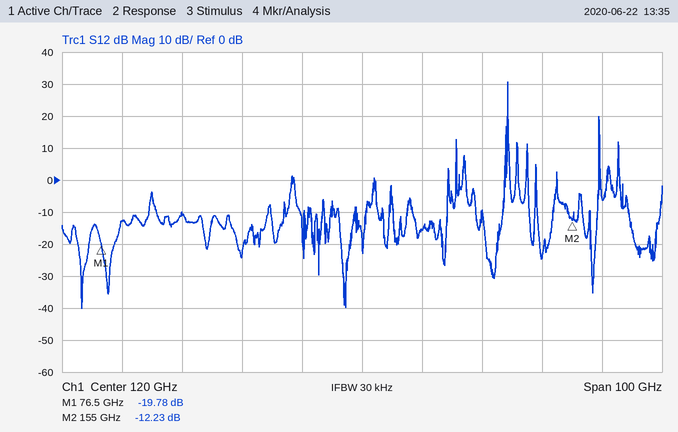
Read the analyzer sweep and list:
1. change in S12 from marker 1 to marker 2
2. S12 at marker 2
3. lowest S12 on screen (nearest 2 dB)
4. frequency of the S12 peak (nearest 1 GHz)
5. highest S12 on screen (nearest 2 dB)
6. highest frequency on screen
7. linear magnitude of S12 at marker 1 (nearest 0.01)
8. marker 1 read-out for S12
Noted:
7.55 dB
-12.23 dB
-40 dB
144 GHz
30 dB
170 GHz
0.10
-19.78 dB
